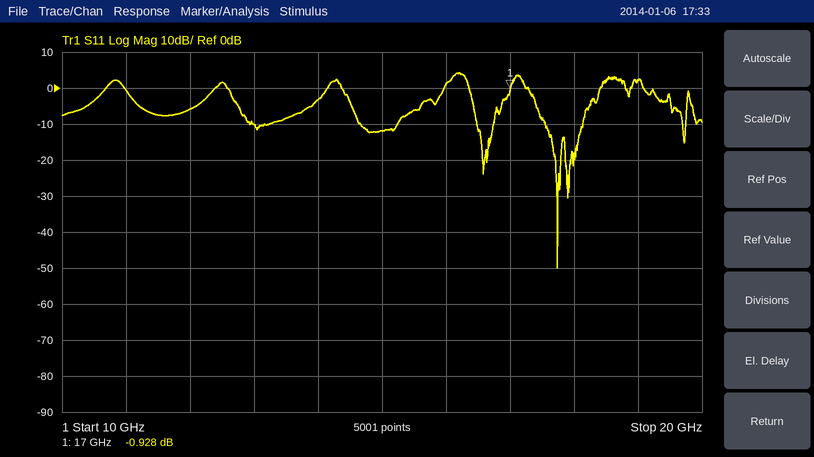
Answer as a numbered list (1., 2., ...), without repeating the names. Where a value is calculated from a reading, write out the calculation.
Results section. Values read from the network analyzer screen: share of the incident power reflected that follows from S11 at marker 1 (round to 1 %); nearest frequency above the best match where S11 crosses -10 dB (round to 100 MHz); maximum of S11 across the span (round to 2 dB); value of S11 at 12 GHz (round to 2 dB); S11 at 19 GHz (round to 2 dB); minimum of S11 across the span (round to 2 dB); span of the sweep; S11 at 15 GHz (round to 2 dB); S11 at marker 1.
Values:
1. 10^(-0.928/10) ≈ 81 %
2. 18.1 GHz
3. 4 dB
4. -6 dB
5. 2 dB
6. -50 dB
7. 10 GHz
8. -12 dB
9. -0.928 dB
